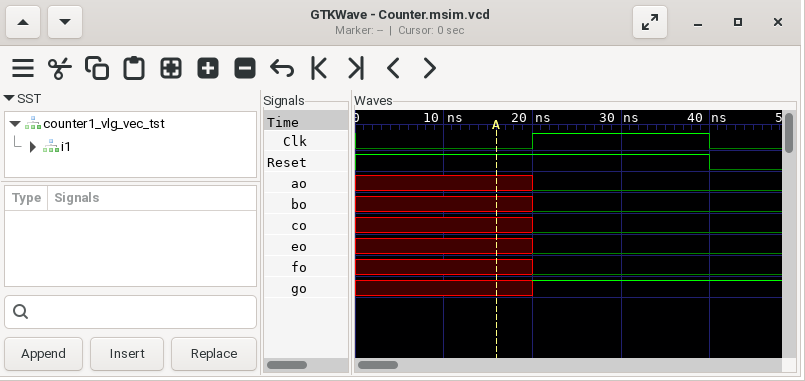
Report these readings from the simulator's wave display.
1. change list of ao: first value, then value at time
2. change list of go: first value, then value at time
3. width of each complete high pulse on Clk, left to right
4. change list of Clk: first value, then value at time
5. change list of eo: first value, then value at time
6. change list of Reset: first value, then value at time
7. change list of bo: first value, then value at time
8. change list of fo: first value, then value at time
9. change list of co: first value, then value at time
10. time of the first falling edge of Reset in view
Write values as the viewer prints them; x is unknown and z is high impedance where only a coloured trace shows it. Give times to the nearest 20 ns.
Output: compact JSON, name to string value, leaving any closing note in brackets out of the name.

{"change list of ao: first value, then value at time": "x, 0 at 20 ns", "change list of go: first value, then value at time": "x, 1 at 20 ns", "width of each complete high pulse on Clk, left to right": "20 ns", "change list of Clk: first value, then value at time": "0, 1 at 20 ns, 0 at 40 ns", "change list of eo: first value, then value at time": "x, 0 at 20 ns", "change list of Reset: first value, then value at time": "1, 0 at 40 ns", "change list of bo: first value, then value at time": "x, 0 at 20 ns", "change list of fo: first value, then value at time": "x, 0 at 20 ns", "change list of co: first value, then value at time": "x, 0 at 20 ns", "time of the first falling edge of Reset in view": "40 ns"}
